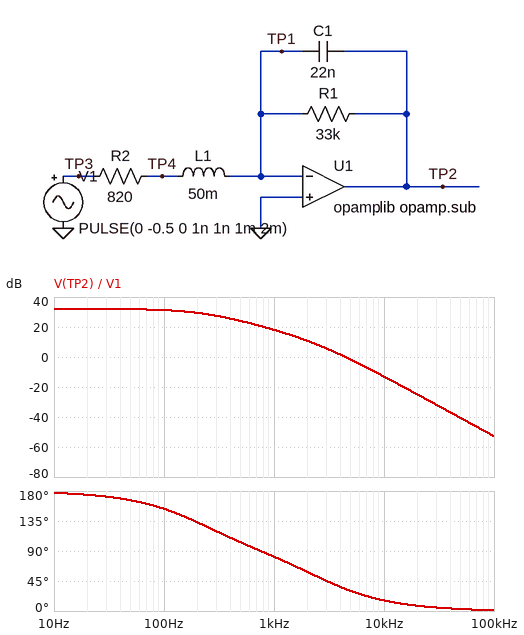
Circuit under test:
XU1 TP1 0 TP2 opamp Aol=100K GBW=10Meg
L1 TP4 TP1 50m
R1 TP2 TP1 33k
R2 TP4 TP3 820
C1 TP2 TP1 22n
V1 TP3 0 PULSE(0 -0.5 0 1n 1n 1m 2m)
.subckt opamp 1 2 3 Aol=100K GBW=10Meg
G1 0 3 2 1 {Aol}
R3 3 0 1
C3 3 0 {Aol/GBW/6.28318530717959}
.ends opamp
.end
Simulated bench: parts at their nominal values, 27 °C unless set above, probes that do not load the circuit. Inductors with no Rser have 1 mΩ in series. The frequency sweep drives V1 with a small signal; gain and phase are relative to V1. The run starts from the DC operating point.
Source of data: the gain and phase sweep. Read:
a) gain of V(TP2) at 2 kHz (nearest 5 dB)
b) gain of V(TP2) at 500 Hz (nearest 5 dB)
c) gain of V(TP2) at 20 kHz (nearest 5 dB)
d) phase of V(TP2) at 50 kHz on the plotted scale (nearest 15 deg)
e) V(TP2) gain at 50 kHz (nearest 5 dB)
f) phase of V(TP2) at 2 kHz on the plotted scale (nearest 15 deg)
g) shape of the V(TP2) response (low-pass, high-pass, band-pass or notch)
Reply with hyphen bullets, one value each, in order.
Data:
- 10 dB
- 25 dB
- -25 dB
- 0 deg
- -40 dB
- 60 deg
- low-pass
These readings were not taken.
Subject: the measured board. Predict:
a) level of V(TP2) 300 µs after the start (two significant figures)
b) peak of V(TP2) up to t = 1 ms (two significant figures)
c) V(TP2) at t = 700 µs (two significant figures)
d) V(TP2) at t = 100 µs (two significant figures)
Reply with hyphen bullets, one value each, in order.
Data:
- 5.6 V
- 15 V
- 12 V
- 1.3 V
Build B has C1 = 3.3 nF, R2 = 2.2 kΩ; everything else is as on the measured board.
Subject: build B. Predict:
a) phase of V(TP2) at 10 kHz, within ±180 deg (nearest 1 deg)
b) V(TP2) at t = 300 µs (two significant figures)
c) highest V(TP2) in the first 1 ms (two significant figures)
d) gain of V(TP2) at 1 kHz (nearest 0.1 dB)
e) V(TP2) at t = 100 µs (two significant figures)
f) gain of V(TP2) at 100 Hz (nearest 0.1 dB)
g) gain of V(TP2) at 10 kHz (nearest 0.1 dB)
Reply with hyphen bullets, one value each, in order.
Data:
- 43 deg
- 6.9 V
- 7.5 V
- 21.8 dB
- 3.7 V
- 23.5 dB
- 1.9 dB
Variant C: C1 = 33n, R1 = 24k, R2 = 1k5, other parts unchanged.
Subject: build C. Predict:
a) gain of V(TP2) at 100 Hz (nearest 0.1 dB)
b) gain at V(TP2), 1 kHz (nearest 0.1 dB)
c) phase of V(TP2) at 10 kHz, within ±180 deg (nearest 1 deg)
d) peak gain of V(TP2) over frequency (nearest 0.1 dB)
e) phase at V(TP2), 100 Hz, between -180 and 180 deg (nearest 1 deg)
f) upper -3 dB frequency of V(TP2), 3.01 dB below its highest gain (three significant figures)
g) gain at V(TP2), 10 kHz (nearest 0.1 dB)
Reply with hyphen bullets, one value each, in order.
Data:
- 23.1 dB
- 9.8 dB
- 27 deg
- 24.1 dB
- 152 deg
- 201 Hz
- -17.2 dB
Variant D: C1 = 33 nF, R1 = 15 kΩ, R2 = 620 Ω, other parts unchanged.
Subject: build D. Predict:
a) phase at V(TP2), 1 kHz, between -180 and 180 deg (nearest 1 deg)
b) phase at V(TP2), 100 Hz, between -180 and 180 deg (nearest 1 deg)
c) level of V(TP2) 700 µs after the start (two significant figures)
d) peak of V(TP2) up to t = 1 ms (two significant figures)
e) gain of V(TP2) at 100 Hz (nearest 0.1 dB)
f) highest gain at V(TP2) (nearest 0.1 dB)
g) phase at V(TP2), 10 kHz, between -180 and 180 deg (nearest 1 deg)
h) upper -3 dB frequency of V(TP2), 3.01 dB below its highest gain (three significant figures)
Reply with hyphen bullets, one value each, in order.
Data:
- 81 deg
- 160 deg
- 8.6 V
- 10 V
- 27.3 dB
- 27.7 dB
- 13 deg
- 313 Hz
